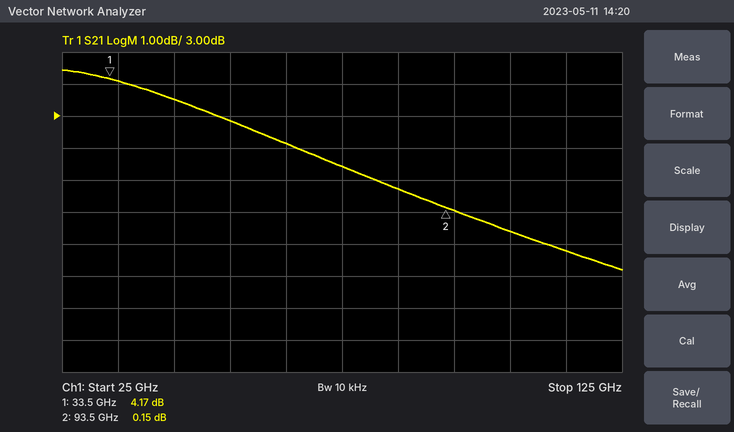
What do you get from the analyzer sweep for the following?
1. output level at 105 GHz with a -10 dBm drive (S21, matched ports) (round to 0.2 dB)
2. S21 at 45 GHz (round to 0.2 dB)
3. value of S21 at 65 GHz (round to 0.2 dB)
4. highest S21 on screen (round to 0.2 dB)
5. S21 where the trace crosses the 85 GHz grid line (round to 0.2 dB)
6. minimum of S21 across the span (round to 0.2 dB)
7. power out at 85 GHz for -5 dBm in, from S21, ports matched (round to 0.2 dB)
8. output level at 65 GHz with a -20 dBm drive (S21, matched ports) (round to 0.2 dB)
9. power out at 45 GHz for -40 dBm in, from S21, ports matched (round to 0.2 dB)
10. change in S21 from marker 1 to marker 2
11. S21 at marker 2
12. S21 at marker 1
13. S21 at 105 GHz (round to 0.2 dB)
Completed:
-10.6 dBm
3.6 dB
2.2 dB
4.4 dB
0.8 dB
-1.8 dB
-4.2 dBm
-17.8 dBm
-36.4 dBm
-4.02 dB
0.15 dB
4.17 dB
-0.6 dB
